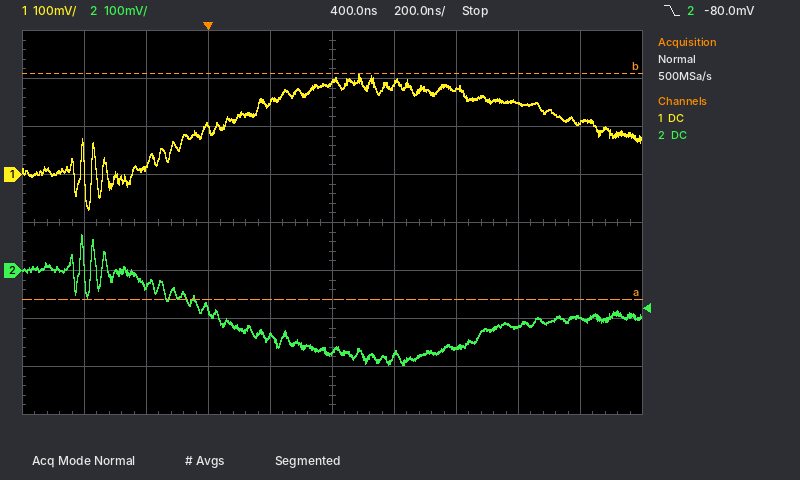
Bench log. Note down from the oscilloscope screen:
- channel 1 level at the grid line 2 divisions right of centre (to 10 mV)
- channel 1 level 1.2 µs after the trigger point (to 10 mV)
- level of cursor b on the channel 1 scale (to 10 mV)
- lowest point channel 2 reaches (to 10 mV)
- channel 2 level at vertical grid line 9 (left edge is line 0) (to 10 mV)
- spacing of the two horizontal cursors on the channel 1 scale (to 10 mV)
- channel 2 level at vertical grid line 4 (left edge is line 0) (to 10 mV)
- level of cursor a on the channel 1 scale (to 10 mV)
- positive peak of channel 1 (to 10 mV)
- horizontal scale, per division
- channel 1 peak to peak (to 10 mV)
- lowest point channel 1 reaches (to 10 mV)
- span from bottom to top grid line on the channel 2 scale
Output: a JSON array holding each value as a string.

["180 mV", "110 mV", "210 mV", "-200 mV", "-100 mV", "470 mV", "-140 mV", "-260 mV", "210 mV", "200 ns", "280 mV", "-70 mV", "800 mV"]
